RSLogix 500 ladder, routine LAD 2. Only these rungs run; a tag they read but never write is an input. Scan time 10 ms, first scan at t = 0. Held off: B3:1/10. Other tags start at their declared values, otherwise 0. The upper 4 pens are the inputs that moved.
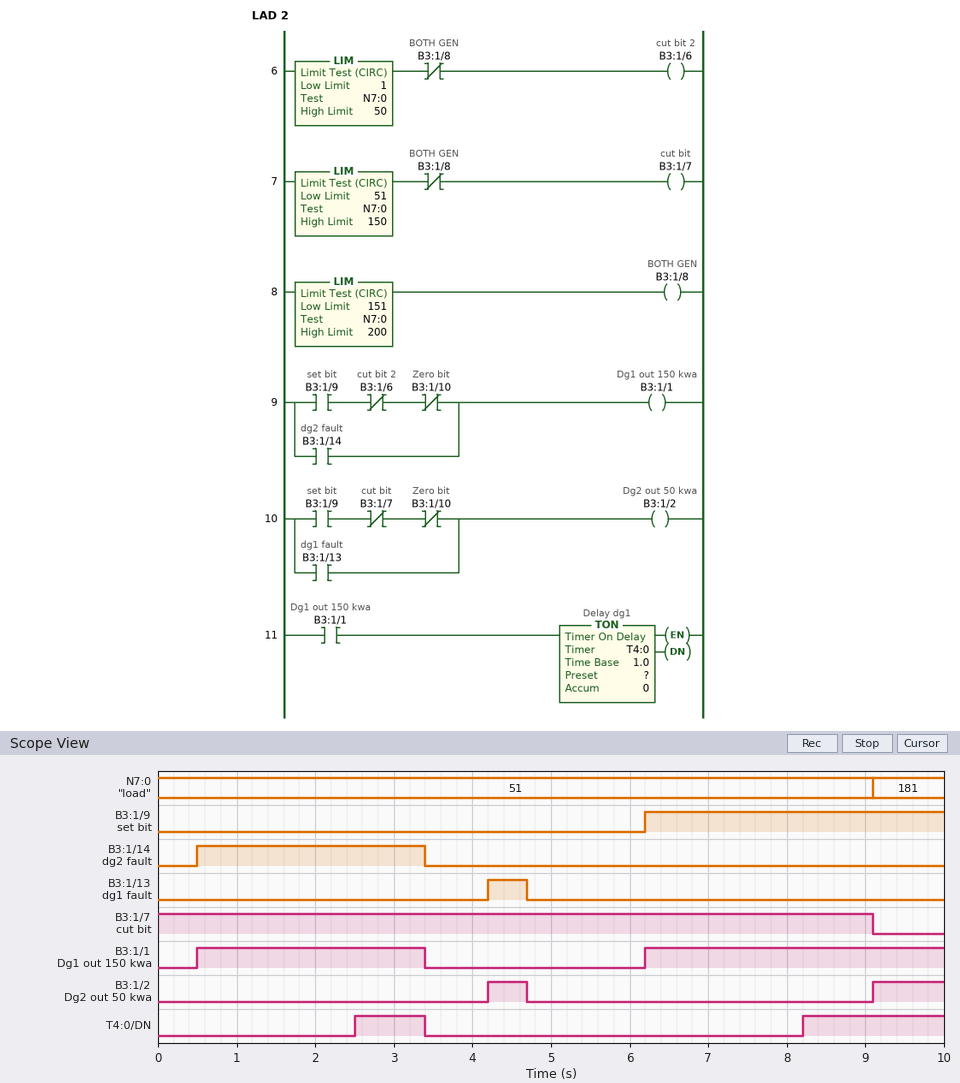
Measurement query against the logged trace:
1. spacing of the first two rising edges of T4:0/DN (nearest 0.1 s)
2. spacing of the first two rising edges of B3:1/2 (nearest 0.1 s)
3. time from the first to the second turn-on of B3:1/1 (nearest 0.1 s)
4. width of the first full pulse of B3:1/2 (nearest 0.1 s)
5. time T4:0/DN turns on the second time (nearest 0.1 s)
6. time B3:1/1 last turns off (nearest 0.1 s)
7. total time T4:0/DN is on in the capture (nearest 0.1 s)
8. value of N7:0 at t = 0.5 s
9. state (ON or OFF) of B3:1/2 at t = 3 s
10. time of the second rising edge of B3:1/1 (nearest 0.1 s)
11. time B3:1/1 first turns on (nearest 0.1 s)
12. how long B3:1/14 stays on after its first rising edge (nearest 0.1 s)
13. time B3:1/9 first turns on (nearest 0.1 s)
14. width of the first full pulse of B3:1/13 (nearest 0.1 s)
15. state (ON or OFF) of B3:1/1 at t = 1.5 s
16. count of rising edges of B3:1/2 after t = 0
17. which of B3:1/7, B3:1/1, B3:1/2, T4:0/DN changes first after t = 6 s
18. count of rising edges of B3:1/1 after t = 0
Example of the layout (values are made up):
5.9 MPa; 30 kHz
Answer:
5.7 s; 4.9 s; 5.7 s; 0.5 s; 8.2 s; 3.4 s; 2.7 s; 51; OFF; 6.2 s; 0.5 s; 2.9 s; 6.2 s; 0.5 s; ON; 2; B3:1/1; 2
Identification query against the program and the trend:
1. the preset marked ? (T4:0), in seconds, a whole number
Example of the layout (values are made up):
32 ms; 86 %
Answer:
2 s
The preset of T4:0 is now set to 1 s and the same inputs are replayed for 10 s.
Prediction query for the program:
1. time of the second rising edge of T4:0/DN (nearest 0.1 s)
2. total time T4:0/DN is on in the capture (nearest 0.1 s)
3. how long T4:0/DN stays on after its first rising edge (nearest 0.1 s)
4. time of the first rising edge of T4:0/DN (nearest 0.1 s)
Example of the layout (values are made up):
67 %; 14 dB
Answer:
7.2 s; 4.7 s; 1.9 s; 1.5 s
